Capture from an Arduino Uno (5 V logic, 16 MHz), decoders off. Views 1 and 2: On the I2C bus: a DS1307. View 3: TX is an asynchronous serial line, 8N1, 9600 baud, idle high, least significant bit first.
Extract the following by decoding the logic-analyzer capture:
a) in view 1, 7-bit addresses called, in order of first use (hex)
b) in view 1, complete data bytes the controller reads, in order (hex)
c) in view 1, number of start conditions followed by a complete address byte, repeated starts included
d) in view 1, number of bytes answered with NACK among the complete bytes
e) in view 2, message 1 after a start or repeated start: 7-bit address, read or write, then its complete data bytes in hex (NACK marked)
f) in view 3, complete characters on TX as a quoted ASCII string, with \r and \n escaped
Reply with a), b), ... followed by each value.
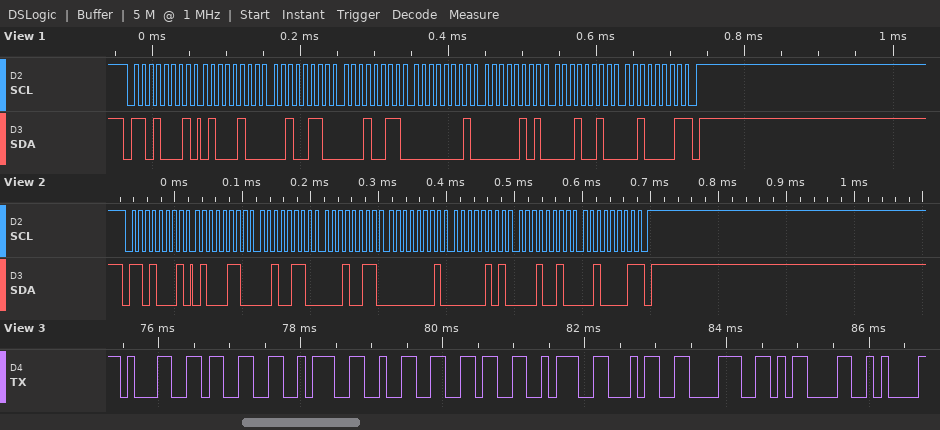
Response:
a) 0x68
b) 44 26 13 01 05 12 21
c) 1
d) 1
e) 0x68 read: 46 26 13 01 05 12 21 NACK
f) "13:26:48\r\n"
